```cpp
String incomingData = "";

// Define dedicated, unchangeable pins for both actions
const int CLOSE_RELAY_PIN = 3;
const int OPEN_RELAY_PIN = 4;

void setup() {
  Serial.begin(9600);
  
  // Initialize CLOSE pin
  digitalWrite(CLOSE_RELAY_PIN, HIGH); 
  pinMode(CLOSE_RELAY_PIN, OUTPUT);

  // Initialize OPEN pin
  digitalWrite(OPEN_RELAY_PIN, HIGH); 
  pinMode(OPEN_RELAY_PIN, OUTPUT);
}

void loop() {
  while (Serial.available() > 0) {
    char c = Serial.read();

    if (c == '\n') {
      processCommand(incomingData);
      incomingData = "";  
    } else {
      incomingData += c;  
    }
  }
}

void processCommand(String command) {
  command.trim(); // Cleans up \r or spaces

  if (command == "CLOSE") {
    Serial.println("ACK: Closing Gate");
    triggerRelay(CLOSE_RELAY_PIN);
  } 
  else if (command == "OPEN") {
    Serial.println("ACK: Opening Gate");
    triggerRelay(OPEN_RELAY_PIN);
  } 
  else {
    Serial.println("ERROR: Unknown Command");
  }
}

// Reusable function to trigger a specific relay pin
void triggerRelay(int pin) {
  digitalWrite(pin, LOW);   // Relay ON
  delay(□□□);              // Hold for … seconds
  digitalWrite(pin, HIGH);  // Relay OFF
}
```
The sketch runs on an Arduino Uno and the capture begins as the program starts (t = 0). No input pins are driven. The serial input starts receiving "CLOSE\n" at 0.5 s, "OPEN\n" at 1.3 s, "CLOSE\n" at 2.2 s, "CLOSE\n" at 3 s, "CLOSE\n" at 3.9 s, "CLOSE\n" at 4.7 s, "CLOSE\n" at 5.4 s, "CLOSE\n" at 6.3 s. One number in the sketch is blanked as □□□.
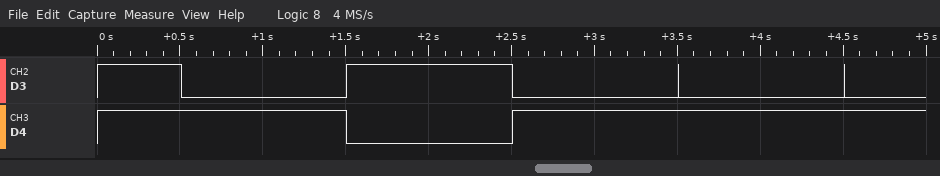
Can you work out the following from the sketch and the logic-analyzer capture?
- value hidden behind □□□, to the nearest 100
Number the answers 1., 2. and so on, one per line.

1. 1000
